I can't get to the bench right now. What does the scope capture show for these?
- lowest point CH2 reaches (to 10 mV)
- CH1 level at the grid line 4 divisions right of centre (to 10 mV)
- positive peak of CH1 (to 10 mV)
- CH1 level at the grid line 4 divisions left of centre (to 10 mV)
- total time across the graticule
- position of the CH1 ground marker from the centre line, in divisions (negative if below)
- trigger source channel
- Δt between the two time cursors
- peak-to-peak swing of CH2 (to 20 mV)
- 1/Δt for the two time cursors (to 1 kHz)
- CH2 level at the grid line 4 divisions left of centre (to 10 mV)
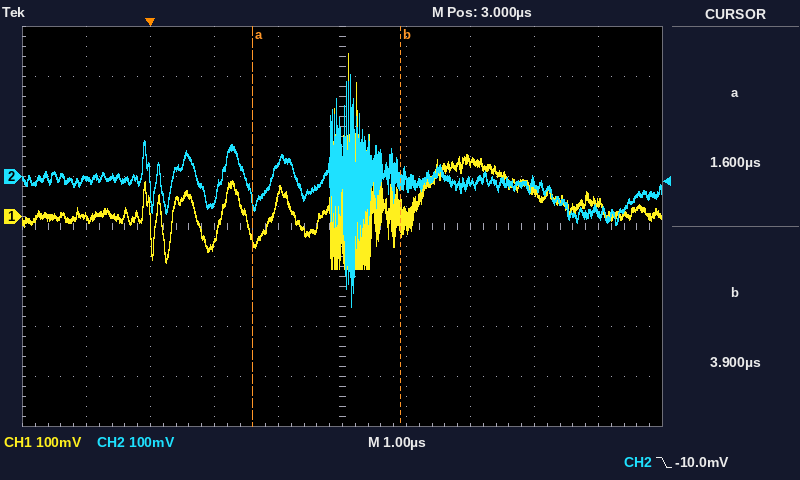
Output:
-260 mV
30 mV
330 mV
0 mV
10 µs
+0.2 div
CH2
2.3 µs
460 mV
435 kHz
0 mV
